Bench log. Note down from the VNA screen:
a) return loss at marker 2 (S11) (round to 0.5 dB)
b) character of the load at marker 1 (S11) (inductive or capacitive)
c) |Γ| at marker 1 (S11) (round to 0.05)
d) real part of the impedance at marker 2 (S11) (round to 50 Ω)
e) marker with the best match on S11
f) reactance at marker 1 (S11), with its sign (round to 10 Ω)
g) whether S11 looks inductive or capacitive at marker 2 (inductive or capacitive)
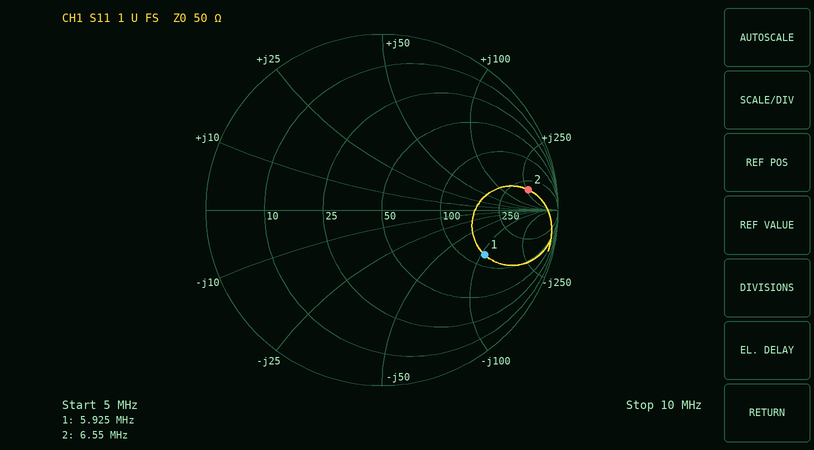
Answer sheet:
1.5 dB
capacitive
0.65
350 Ω
marker 1
-110 Ω
inductive
